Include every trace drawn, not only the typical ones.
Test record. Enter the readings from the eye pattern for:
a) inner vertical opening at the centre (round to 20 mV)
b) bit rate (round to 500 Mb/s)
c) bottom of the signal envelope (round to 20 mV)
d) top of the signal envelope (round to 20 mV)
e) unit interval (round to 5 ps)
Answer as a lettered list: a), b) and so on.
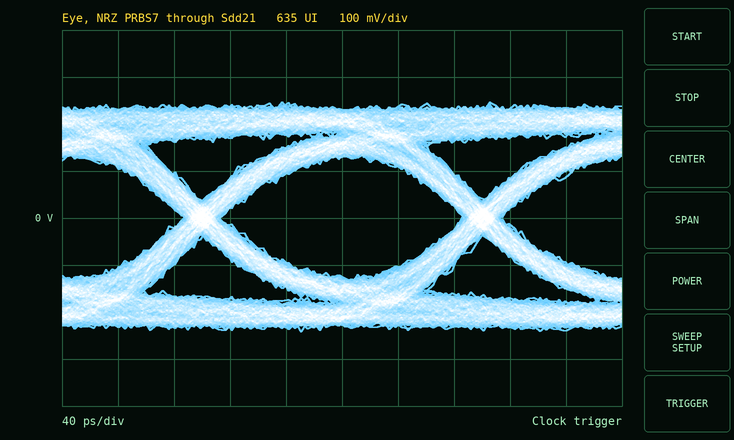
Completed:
a) 260 mV
b) 5.0 Gb/s
c) -240 mV
d) 240 mV
e) 200 ps
